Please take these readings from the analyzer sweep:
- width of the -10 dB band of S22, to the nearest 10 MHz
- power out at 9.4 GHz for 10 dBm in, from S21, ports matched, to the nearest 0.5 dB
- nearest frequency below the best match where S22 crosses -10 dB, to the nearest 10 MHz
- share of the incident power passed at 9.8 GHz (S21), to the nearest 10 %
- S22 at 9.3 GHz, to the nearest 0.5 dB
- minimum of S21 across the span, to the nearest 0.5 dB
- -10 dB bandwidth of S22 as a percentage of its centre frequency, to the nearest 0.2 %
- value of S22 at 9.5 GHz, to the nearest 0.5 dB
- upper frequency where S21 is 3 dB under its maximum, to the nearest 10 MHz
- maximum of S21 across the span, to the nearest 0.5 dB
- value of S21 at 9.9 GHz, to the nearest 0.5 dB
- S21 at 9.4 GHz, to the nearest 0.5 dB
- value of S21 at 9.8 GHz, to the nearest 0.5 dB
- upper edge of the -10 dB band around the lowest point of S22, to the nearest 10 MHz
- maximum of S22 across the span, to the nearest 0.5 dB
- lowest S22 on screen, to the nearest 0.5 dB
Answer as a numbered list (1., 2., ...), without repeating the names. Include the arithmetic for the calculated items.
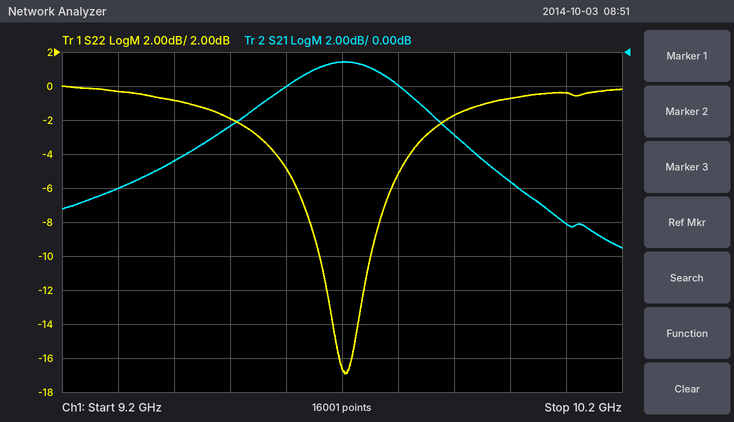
1. 9.75 GHz − 9.66 GHz = 90 MHz
2. 10 dBm + (-6.5 dB) = 3.5 dBm
3. 9.66 GHz
4. 10^(-2/10) ≈ 63.1 %, so 60 % to the nearest 10 %
5. -0.5 dB
6. -11.5 dB
7. 90 MHz / 9.705 GHz ≈ 0.927 %, so 1.0 % to the nearest 0.2 %
8. -2.0 dB
9. 9.86 GHz
10. -0.5 dB
11. -5.0 dB
12. -6.5 dB
13. -2.0 dB
14. 9.75 GHz
15. 0.0 dB
16. -17.0 dB
